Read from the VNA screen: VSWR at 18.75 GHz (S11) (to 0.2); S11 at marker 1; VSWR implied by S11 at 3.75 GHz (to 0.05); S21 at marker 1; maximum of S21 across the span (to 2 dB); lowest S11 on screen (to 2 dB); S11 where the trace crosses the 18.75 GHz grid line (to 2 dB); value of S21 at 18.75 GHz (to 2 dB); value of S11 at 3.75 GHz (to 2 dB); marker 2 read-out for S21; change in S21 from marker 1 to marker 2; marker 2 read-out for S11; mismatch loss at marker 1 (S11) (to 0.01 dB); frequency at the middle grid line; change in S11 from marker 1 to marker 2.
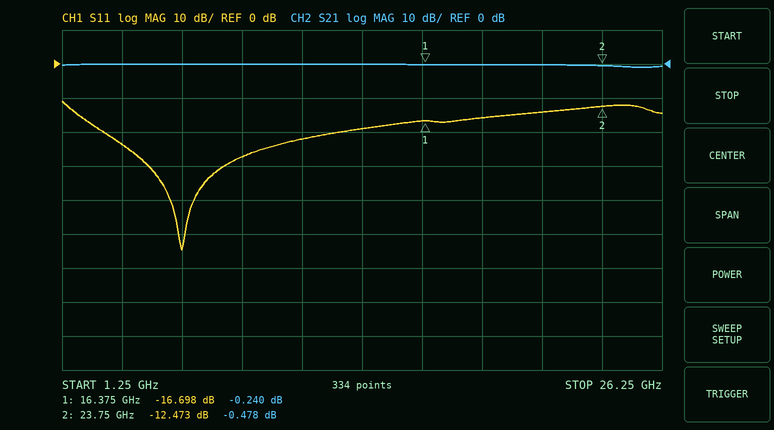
1.4
-16.698 dB
1.15
-0.240 dB
0 dB
-54 dB
-16 dB
0 dB
-24 dB
-0.478 dB
-0.238 dB
-12.473 dB
0.09 dB
13.75 GHz
4.225 dB
